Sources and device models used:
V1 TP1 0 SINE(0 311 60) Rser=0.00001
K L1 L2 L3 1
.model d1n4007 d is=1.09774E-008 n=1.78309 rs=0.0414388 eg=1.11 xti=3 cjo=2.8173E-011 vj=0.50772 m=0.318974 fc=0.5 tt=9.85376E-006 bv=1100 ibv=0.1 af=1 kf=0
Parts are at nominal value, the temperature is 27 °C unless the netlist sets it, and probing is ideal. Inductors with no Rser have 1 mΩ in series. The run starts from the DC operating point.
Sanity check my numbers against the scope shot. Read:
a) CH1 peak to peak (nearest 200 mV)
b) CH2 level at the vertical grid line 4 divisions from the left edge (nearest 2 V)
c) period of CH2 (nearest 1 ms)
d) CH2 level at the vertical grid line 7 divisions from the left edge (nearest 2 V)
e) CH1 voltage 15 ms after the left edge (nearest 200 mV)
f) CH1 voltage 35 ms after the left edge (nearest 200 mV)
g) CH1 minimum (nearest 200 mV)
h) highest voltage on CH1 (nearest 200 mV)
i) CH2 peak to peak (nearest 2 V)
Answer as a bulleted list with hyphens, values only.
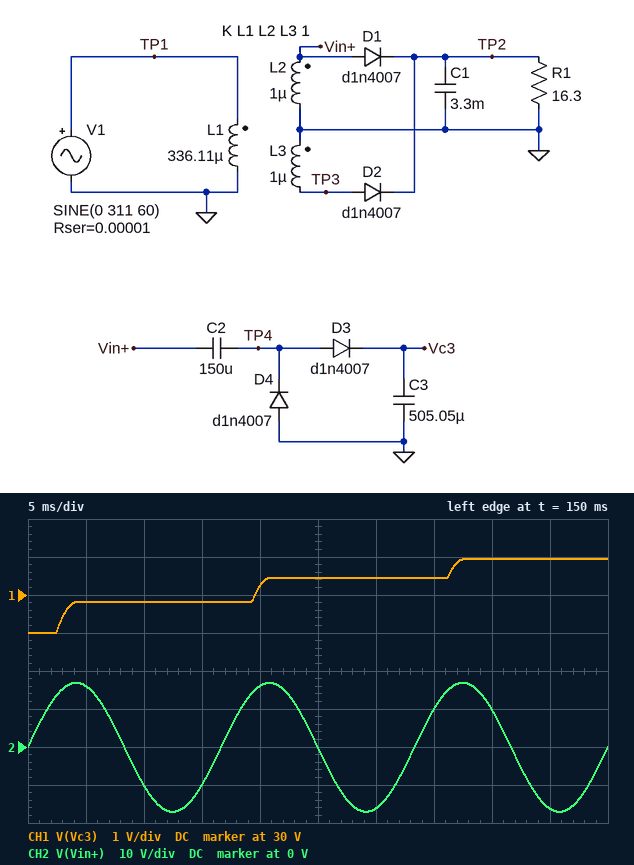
- 2.0 V
- 16 V
- 17 ms
- 10 V
- 29.8 V
- 30.4 V
- 29.0 V
- 31.0 V
- 34 V
